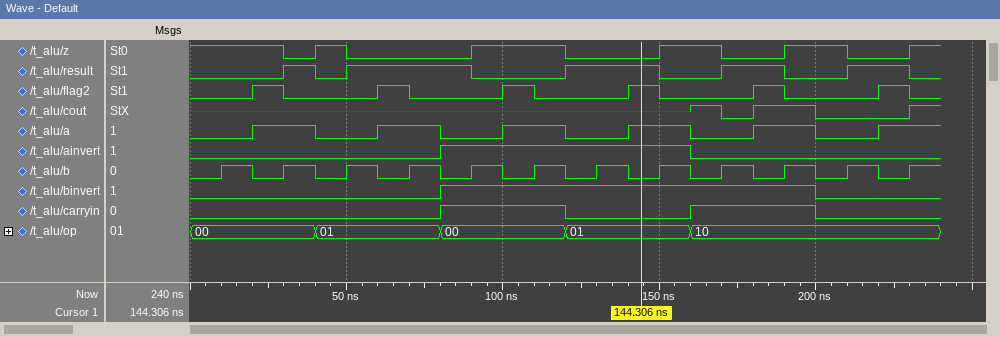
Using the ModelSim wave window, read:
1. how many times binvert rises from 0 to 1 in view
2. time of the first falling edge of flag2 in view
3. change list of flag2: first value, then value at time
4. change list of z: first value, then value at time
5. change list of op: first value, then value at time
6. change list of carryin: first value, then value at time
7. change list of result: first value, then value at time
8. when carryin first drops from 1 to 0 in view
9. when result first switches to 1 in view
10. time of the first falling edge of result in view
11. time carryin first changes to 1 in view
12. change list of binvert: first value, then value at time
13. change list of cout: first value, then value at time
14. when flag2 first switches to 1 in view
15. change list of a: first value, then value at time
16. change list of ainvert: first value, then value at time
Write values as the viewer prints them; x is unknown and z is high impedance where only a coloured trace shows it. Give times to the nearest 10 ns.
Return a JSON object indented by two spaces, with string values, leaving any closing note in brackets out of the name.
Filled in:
{
  "how many times binvert rises from 0 to 1 in view": "1",
  "time of the first falling edge of flag2 in view": "30 ns",
  "change list of flag2: first value, then value at time": "0, 1 at 20 ns, 0 at 30 ns, 1 at 60 ns, 0 at 70 ns, 1 at 100 ns, 0 at 110 ns, 1 at 140 ns, 0 at 150 ns, 1 at 180 ns, 0 at 190 ns, 1 at 220 ns, 0 at 230 ns",
  "change list of z: first value, then value at time": "1, 0 at 30 ns, 1 at 40 ns, 0 at 50 ns, 1 at 90 ns, 0 at 120 ns, 1 at 150 ns, 0 at 170 ns, 1 at 190 ns, 0 at 210 ns, 1 at 230 ns",
  "change list of op: first value, then value at time": "00, 01 at 40 ns, 00 at 80 ns, 01 at 120 ns, 10 at 160 ns",
  "change list of carryin: first value, then value at time": "0, 1 at 80 ns, 0 at 120 ns, 1 at 160 ns, 0 at 200 ns",
  "change list of result: first value, then value at time": "0, 1 at 30 ns, 0 at 40 ns, 1 at 50 ns, 0 at 90 ns, 1 at 120 ns, 0 at 150 ns, 1 at 170 ns, 0 at 190 ns, 1 at 210 ns, 0 at 230 ns",
  "when carryin first drops from 1 to 0 in view": "120 ns",
  "when result first switches to 1 in view": "30 ns",
  "time of the first falling edge of result in view": "40 ns",
  "time carryin first changes to 1 in view": "80 ns",
  "change list of binvert: first value, then value at time": "0, 1 at 80 ns, 0 at 200 ns",
  "change list of cout: first value, then value at time": "x, 1 at 160 ns, 0 at 170 ns, 1 at 180 ns, 0 at 200 ns, 1 at 230 ns",
  "when flag2 first switches to 1 in view": "20 ns",
  "change list of a: first value, then value at time": "0, 1 at 20 ns, 0 at 40 ns, 1 at 60 ns, 0 at 80 ns, 1 at 100 ns, 0 at 120 ns, 1 at 140 ns, 0 at 160 ns, 1 at 180 ns, 0 at 200 ns, 1 at 220 ns",
  "change list of ainvert: first value, then value at time": "0, 1 at 80 ns, 0 at 160 ns"
}
